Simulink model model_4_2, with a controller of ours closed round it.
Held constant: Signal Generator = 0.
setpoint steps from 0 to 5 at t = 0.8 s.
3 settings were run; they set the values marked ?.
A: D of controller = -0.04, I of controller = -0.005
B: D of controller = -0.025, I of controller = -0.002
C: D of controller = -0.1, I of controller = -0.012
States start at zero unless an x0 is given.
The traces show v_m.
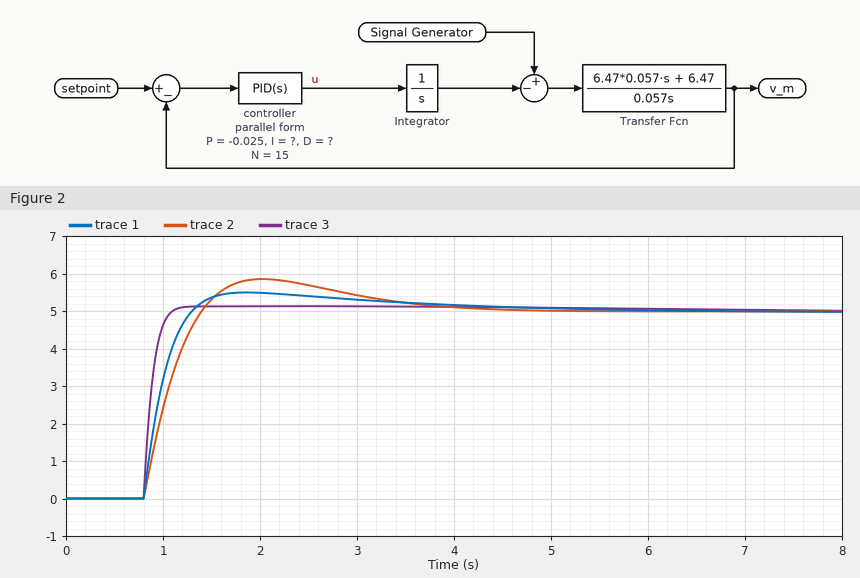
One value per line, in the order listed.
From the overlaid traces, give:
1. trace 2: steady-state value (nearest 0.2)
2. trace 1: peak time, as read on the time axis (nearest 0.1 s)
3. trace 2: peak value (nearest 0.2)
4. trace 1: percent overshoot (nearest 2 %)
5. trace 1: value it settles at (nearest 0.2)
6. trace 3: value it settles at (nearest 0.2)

5.0
1.9 s
5.8
10 %
5.0
5.0
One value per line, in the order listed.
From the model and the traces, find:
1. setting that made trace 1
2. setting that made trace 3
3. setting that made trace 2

A
C
B
